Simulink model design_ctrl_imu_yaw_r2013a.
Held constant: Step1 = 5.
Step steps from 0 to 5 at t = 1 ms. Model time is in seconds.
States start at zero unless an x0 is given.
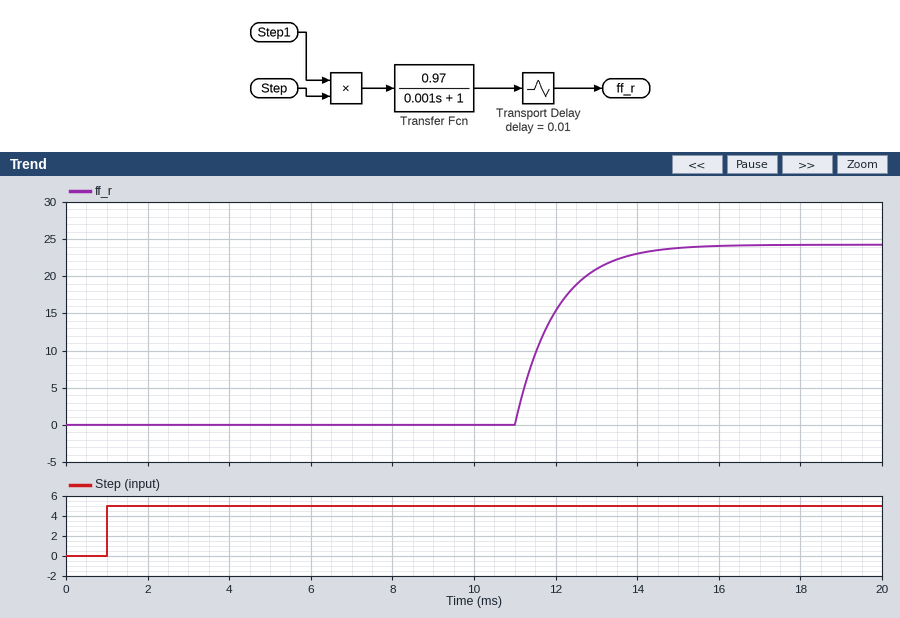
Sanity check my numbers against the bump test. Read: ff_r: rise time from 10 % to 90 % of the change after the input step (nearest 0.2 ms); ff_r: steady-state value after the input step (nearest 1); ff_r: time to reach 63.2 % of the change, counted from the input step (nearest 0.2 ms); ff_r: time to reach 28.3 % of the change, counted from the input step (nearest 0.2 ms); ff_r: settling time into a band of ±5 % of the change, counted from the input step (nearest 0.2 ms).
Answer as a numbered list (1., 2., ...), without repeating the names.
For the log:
1. 2.2 ms
2. 24
3. 11.0 ms
4. 10.4 ms
5. 13.0 ms
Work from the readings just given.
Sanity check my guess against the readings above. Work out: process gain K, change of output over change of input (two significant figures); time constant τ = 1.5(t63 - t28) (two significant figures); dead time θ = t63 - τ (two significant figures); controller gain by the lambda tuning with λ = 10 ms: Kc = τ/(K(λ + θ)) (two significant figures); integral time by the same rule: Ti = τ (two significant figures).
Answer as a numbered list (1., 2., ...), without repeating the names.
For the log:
1. 4.8
2. 0.90 ms
3. 10 ms
4. 0.0094
5. 0.90 ms
